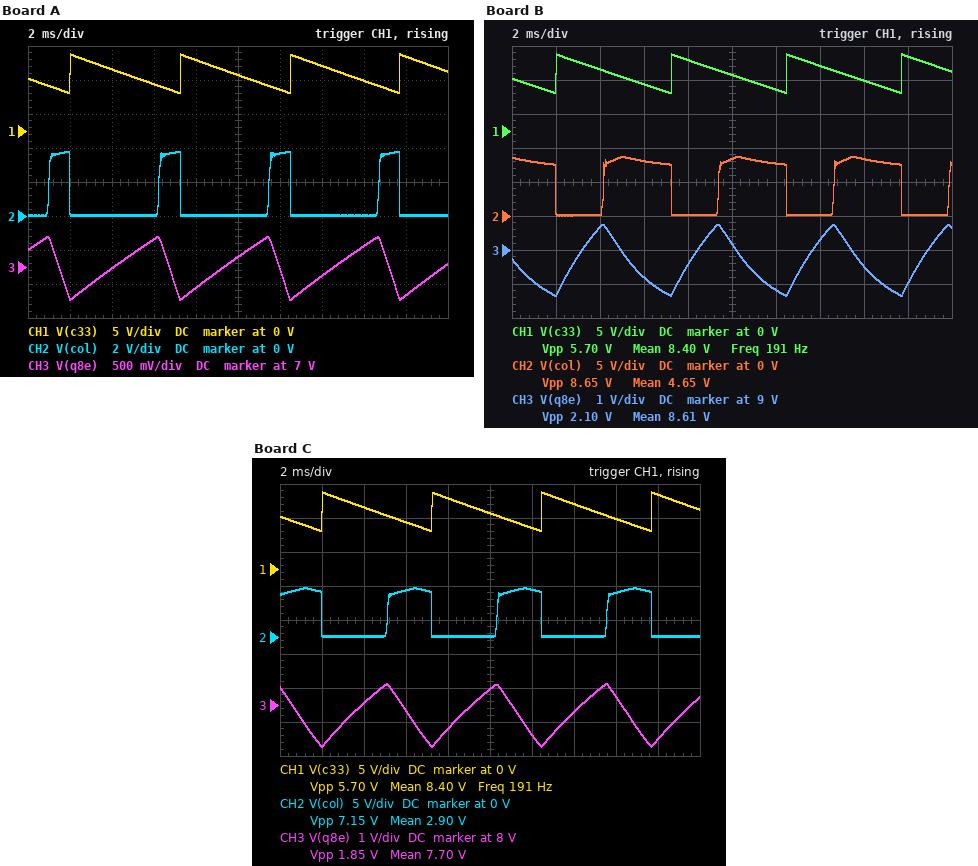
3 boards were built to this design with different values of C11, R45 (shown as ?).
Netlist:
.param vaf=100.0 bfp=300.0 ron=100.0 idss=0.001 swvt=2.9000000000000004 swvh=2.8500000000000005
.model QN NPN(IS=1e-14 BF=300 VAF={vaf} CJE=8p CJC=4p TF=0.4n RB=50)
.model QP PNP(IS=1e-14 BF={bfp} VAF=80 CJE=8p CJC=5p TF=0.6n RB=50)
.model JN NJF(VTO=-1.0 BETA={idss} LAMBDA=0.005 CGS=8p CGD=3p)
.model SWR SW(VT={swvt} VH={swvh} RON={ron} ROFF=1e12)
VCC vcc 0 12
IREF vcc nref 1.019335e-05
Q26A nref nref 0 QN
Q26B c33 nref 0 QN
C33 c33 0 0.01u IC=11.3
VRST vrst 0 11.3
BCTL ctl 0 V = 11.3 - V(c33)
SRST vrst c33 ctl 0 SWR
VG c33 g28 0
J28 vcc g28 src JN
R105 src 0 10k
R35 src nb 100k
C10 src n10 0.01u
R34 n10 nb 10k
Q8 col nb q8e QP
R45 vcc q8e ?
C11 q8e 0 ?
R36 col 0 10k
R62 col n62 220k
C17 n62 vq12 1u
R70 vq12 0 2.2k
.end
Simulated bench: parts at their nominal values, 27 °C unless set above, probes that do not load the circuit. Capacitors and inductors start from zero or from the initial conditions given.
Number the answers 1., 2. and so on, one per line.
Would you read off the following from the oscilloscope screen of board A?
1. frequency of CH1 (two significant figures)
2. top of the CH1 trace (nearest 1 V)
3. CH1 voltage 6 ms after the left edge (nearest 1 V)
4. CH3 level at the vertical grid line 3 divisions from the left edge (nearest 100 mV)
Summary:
1. 190 Hz
2. 11 V
3. 7 V
4. 7.4 V
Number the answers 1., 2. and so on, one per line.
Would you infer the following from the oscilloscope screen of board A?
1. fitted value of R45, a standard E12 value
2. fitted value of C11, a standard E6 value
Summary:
1. 68 kΩ
2. 330 nF
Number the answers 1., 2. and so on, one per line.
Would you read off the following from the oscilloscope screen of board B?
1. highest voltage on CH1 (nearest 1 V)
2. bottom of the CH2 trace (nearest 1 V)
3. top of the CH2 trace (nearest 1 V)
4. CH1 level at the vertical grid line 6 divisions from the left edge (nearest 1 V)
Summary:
1. 11 V
2. 0 V
3. 9 V
4. 6 V
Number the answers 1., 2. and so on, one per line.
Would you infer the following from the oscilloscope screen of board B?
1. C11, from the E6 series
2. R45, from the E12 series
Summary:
1. 470 nF
2. 6.8 kΩ
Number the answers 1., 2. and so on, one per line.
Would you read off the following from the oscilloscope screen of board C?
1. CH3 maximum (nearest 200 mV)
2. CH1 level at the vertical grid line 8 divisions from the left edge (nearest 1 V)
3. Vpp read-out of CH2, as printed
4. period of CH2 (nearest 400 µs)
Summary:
1. 8.6 V
2. 7 V
3. 7.15 V
4. 5.2 ms
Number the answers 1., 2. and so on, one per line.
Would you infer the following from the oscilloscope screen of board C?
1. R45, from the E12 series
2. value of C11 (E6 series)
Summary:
1. 15 kΩ
2. 470 nF
